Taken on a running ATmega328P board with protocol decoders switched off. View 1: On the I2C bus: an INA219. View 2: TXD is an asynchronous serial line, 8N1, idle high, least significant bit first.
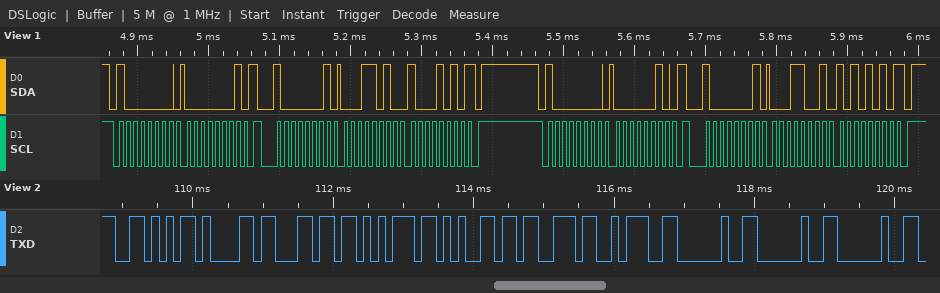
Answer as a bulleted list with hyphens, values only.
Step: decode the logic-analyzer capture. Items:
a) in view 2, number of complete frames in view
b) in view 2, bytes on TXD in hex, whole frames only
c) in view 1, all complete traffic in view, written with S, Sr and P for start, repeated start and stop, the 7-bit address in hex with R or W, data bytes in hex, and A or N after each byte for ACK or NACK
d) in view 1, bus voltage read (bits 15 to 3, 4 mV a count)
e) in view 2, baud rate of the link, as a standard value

- 10
- 56 61 6C 75 65 73 3A 20 20 20
- S 40W A 01 A Sr 40R A 1A A 8A N P S 40W A 02 A Sr 40R A 19 A AA N P
- 3.284 V
- 9600 baud
